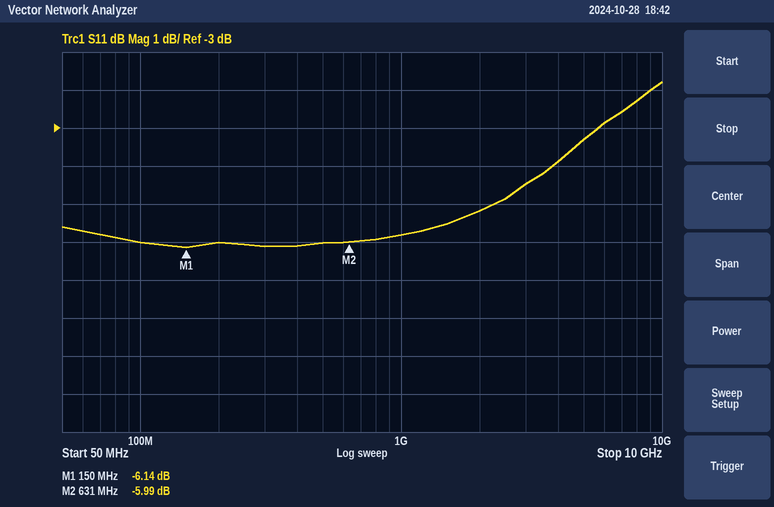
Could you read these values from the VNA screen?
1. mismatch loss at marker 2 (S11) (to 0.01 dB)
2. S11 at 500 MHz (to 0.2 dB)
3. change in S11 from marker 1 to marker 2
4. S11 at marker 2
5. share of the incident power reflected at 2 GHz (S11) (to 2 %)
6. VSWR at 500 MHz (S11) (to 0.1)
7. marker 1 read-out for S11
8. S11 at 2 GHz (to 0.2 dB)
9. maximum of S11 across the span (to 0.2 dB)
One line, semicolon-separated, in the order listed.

1.26 dB; -6.0 dB; 0.15 dB; -5.99 dB; 30 %; 3.0; -6.14 dB; -5.2 dB; -1.8 dB
